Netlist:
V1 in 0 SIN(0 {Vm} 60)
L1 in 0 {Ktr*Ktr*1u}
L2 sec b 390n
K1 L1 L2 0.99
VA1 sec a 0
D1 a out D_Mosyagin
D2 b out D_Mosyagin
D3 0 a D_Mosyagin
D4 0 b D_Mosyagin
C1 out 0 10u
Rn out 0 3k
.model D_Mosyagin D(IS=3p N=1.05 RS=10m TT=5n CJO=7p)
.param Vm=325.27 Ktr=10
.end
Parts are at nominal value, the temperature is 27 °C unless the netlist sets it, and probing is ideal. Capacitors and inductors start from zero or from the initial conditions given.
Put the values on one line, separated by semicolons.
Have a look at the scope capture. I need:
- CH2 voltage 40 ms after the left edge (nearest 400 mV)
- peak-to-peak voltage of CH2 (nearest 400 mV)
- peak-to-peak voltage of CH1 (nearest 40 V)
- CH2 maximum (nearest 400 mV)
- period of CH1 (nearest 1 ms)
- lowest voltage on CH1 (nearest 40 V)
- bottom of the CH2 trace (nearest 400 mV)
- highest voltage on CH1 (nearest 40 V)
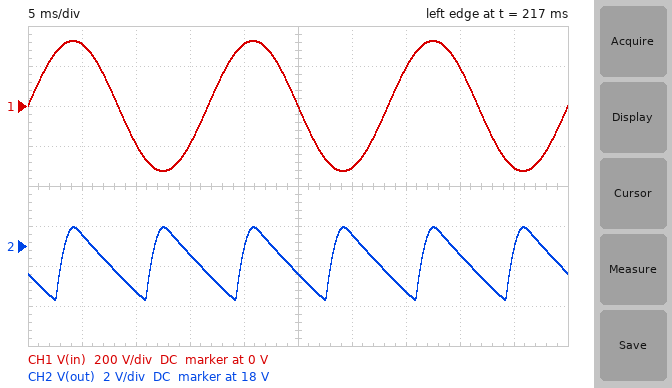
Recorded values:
17.6 V; 3.6 V; 640 V; 18.8 V; 17 ms; -320 V; 15.2 V; 320 V
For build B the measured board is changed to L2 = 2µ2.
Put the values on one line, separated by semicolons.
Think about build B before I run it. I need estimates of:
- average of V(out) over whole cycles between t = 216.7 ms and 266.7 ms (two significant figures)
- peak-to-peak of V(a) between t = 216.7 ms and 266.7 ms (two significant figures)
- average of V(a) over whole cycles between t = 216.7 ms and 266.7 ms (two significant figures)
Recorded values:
42 V; 48 V; 21 V
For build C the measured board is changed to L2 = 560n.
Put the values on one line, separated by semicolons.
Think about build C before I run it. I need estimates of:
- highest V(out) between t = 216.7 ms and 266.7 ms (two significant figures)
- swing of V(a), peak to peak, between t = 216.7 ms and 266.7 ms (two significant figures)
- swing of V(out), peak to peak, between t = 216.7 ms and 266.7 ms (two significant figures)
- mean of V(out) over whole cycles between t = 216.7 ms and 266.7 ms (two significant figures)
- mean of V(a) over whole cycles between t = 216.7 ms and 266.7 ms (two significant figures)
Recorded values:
23 V; 24 V; 4.4 V; 21 V; 10 V
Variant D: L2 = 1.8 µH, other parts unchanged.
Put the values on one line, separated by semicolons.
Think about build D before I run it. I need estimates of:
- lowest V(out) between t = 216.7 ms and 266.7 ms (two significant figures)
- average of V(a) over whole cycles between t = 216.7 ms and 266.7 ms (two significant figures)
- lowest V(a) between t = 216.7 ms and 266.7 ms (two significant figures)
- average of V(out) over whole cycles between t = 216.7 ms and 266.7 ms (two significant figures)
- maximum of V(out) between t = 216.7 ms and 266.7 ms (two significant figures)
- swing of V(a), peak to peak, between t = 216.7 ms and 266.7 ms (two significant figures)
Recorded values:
34 V; 19 V; -660 mV; 38 V; 42 V; 43 V
